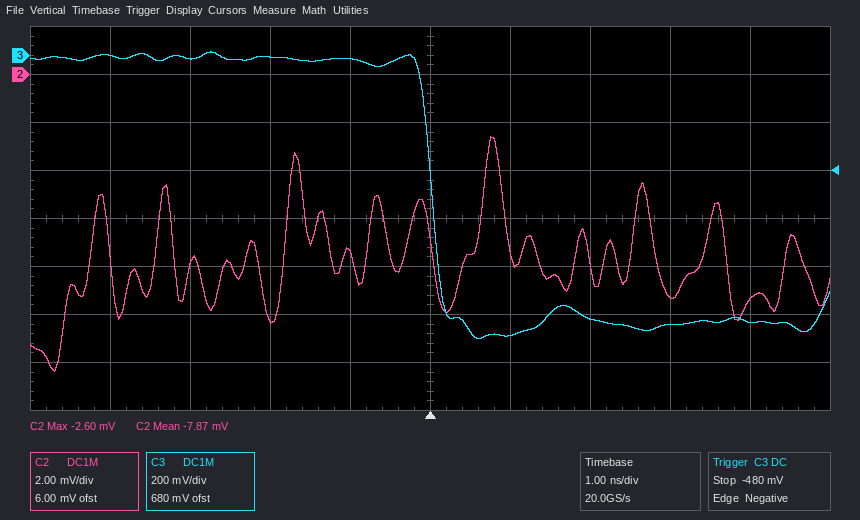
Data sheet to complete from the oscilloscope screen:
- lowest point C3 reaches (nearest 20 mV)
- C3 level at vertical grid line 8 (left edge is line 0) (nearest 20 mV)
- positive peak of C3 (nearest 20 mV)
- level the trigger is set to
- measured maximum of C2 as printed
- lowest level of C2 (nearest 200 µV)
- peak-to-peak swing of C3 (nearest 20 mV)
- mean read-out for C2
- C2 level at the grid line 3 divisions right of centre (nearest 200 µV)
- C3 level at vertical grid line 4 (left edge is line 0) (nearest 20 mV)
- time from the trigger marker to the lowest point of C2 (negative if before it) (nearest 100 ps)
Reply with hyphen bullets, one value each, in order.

- -1.18 V
- -1.12 V
- 20 mV
- -480 mV
- -2.60 mV
- -12.4 mV
- 1.20 V
- -7.87 mV
- -9.2 mV
- -20 mV
- -4.7 ns
